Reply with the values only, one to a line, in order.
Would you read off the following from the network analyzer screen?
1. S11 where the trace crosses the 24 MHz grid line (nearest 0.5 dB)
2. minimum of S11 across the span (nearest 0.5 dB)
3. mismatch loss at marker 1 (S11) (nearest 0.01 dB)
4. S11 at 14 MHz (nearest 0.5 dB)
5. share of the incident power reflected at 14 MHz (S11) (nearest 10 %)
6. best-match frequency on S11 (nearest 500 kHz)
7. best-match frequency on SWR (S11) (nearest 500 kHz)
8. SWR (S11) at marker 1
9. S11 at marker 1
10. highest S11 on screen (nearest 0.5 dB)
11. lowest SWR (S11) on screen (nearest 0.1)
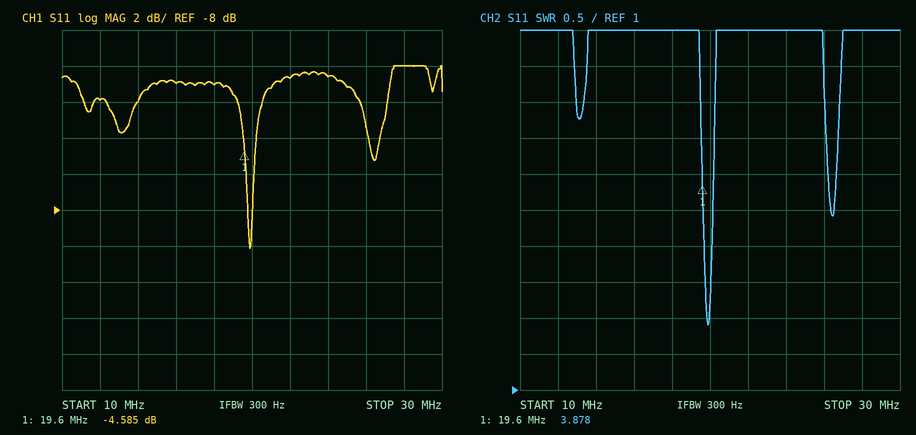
-0.5 dB
-10.0 dB
1.86 dB
-2.0 dB
60 %
20.0 MHz
20.0 MHz
3.878
-4.585 dB
0.0 dB
1.9
